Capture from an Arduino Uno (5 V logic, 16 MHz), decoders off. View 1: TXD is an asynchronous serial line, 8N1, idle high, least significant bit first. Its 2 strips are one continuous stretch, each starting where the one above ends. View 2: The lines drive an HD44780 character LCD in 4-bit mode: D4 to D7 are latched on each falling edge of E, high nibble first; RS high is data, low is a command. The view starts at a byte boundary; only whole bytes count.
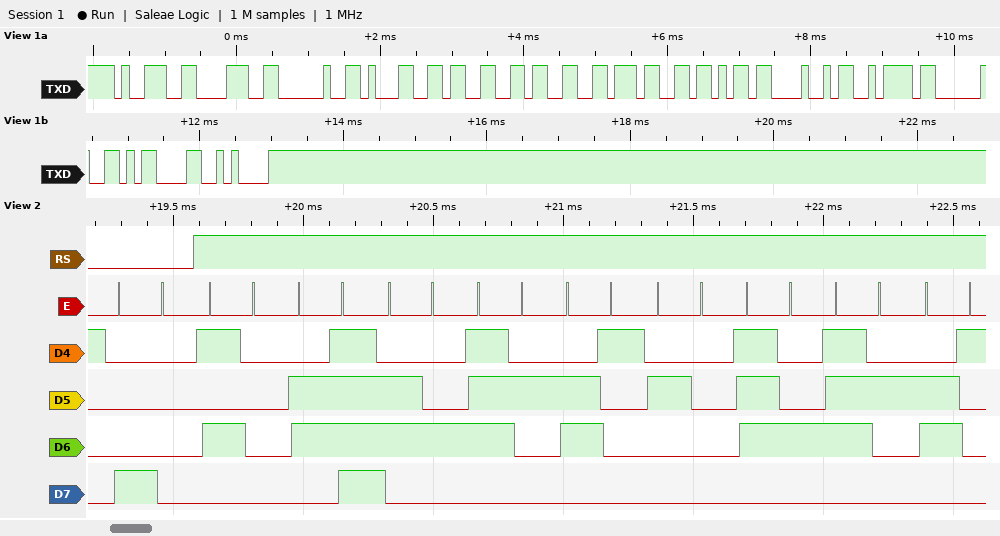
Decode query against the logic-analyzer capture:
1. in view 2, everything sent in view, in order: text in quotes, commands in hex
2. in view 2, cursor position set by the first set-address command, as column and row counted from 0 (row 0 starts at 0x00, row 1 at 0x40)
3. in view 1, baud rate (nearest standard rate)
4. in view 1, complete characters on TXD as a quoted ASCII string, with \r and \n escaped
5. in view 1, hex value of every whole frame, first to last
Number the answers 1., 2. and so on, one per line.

1. 0x80 "Podra tra"
2. column 0, row 0
3. 9600 baud
4. "98 1337kHz \r\n"
5. 39 38 20 31 33 33 37 6B 48 7A 20 0D 0A
